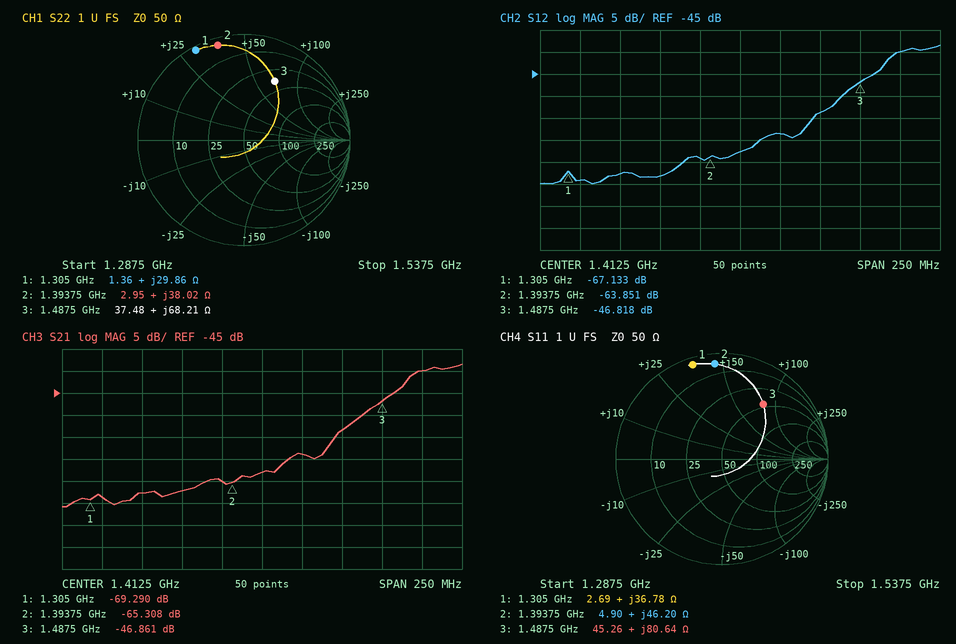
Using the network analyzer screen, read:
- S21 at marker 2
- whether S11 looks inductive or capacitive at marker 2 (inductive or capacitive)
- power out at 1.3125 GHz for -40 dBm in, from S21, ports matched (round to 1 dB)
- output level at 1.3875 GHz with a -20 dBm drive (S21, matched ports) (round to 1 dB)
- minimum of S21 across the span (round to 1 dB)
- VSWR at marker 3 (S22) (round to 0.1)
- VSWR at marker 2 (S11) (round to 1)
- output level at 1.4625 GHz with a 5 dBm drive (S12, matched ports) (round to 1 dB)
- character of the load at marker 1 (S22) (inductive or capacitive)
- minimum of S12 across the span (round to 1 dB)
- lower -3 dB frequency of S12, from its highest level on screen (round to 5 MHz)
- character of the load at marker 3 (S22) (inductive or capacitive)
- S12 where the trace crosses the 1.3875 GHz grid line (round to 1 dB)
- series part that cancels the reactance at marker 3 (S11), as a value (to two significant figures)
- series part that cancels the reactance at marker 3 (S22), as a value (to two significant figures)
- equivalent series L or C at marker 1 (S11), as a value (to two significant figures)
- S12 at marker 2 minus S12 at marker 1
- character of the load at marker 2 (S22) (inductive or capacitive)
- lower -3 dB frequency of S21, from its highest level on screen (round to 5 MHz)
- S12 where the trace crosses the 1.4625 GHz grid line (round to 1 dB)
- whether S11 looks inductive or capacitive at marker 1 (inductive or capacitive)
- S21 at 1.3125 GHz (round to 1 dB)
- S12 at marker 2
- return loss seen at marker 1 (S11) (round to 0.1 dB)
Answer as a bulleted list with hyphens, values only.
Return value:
- -65.308 dB
- inductive
- -109 dBm
- -85 dBm
- -71 dB
- 4.3
- 19
- -49 dBm
- inductive
- -70 dB
- 1.505 GHz
- inductive
- -64 dB
- 1.3 pF
- 1.6 pF
- 4.5 nH
- 3.282 dB
- inductive
- 1.505 GHz
- -54 dB
- inductive
- -69 dB
- -63.851 dB
- 0.6 dB
